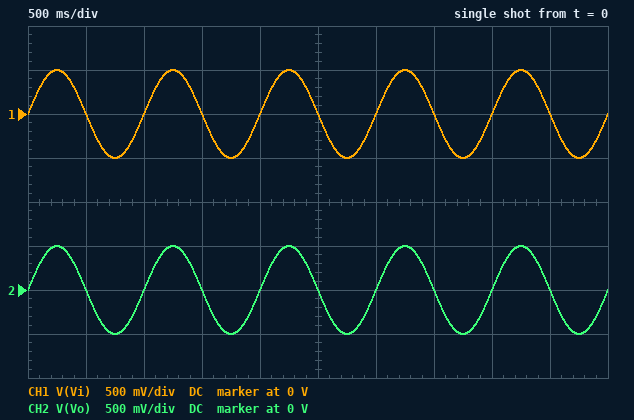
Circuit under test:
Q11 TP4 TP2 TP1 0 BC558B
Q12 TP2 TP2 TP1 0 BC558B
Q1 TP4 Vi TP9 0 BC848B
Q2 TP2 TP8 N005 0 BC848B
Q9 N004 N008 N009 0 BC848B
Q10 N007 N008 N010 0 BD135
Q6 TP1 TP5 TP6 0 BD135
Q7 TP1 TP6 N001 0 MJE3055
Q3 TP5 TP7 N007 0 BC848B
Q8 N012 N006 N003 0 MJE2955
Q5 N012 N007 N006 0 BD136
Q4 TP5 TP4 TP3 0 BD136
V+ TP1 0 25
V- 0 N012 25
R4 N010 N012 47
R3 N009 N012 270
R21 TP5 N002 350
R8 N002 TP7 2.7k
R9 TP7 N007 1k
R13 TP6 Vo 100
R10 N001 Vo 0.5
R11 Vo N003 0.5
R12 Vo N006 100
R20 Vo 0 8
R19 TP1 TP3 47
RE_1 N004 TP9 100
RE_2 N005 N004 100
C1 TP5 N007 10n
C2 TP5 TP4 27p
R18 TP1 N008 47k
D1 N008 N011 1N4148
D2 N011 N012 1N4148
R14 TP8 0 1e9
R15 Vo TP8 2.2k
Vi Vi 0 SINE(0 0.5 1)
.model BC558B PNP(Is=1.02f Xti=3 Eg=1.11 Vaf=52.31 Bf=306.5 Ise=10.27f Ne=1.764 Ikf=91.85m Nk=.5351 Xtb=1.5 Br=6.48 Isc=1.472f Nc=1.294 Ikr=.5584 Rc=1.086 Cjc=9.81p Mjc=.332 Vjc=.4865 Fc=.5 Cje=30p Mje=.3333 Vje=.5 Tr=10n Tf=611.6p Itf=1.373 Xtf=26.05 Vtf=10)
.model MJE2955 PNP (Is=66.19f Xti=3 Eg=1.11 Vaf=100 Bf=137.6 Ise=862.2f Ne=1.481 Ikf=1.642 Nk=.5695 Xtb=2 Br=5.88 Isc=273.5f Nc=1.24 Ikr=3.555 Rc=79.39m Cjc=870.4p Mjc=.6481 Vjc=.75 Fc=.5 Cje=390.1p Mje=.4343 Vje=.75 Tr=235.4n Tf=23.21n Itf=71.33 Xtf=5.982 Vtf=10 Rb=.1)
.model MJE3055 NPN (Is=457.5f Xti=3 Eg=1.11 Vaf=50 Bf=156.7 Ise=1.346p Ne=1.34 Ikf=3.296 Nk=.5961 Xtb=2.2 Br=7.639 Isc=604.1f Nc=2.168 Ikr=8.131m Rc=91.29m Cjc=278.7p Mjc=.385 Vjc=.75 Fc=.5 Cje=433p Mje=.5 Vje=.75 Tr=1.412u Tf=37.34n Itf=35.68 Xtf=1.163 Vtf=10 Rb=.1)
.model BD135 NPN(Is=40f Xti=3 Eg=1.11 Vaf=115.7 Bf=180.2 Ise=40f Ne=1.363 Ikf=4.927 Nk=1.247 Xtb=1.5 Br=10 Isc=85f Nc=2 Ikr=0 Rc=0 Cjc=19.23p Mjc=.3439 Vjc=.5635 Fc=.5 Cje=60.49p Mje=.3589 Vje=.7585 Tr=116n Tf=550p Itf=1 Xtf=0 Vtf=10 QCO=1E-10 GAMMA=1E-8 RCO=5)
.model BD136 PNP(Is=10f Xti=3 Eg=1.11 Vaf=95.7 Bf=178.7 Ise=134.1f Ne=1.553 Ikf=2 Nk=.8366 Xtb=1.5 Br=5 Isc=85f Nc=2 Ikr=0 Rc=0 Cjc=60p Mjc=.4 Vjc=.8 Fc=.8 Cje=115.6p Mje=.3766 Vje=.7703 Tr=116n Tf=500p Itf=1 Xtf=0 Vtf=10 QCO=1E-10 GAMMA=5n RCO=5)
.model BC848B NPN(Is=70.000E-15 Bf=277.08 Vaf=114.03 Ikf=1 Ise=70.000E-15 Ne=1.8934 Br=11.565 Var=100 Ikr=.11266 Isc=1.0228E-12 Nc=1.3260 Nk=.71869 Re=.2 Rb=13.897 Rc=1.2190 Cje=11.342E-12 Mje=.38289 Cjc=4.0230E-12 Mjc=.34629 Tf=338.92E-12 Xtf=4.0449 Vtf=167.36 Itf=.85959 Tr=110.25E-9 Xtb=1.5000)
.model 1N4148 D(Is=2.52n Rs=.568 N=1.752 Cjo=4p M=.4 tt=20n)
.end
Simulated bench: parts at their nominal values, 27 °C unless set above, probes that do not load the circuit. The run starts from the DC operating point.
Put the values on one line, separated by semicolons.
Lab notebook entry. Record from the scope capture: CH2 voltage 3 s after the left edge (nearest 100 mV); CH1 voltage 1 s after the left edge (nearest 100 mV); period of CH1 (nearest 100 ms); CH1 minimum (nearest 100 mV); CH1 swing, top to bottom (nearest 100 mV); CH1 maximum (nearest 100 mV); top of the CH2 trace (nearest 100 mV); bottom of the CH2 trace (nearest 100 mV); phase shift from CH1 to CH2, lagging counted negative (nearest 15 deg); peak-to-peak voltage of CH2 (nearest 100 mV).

0 V; 0 V; 1.0 s; -500 mV; 1.0 V; 500 mV; 500 mV; -500 mV; 0 deg; 1.0 V
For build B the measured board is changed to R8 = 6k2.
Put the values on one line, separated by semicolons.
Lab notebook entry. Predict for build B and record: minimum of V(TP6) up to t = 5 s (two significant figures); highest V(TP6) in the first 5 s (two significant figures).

1.3 V; 2.4 V
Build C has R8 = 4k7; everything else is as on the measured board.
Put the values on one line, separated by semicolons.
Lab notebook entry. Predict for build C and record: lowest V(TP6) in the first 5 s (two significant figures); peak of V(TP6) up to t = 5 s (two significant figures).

830 mV; 1.9 V
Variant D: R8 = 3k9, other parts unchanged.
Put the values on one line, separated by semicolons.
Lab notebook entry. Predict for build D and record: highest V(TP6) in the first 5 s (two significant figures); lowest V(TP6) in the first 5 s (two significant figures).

1.6 V; 570 mV
